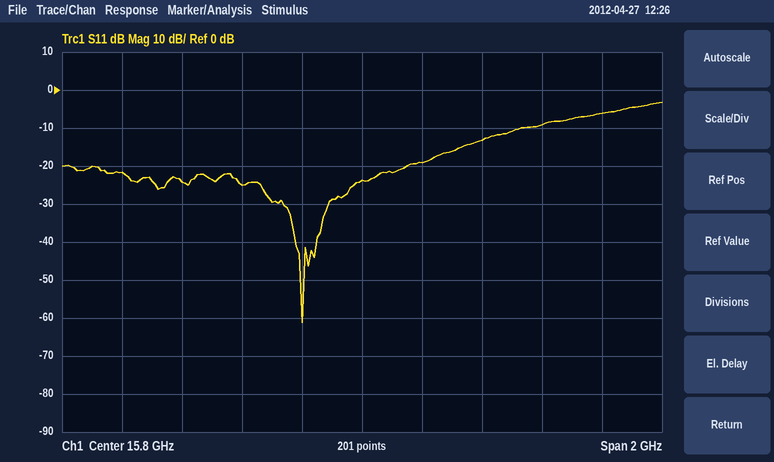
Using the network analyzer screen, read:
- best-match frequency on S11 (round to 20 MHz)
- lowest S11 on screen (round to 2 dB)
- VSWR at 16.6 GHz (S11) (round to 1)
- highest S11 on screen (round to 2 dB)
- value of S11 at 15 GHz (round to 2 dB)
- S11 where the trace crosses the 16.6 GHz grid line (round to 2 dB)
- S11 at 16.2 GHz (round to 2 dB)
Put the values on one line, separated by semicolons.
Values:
15.60 GHz; -62 dB; 3; -4 dB; -22 dB; -6 dB; -14 dB
